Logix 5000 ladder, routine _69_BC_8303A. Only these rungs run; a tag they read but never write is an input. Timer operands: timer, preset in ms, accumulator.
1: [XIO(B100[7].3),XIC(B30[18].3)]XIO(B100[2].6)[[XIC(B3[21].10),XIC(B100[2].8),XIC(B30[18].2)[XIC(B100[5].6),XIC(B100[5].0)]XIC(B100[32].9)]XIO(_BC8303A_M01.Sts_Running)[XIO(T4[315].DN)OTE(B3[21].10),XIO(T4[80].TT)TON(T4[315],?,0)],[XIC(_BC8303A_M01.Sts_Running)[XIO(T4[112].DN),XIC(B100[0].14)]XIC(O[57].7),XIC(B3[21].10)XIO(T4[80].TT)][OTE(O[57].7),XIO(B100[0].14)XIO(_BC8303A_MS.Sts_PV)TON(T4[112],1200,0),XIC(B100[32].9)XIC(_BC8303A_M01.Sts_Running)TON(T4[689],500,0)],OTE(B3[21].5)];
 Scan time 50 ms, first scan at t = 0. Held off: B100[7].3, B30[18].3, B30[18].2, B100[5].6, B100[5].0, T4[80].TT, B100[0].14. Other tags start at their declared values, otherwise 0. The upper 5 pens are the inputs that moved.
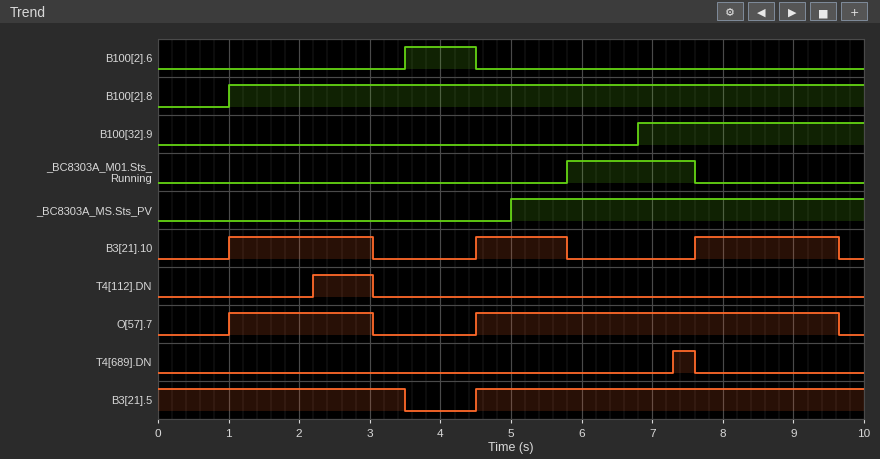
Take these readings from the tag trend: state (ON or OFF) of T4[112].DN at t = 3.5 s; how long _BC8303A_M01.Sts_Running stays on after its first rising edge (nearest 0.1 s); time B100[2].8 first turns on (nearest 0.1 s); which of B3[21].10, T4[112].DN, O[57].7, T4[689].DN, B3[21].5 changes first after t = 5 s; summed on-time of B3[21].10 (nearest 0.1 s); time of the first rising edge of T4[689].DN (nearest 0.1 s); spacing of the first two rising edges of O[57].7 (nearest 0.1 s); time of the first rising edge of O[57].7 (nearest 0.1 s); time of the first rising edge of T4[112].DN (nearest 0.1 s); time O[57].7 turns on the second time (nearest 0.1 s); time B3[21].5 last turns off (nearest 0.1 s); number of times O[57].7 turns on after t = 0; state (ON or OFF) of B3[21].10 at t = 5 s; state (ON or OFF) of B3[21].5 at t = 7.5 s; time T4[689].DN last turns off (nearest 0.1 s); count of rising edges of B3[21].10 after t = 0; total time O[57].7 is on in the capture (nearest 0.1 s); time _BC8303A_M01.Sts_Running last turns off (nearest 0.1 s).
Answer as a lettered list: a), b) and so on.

a) OFF
b) 1.8 s
c) 1.0 s
d) B3[21].10
e) 5.4 s
f) 7.3 s
g) 3.5 s
h) 1.0 s
i) 2.2 s
j) 4.5 s
k) 3.5 s
l) 2
m) ON
n) ON
o) 7.6 s
p) 3
q) 7.2 s
r) 7.6 s
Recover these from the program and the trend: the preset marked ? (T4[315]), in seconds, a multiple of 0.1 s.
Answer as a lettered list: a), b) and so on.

a) 2.0 s
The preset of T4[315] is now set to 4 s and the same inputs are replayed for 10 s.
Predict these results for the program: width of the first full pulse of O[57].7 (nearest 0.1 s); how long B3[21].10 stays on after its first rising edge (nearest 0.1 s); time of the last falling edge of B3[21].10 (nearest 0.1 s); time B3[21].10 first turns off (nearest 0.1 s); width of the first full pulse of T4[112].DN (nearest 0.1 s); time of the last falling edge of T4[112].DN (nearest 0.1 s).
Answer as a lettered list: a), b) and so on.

a) 2.5 s
b) 2.5 s
c) 5.8 s
d) 3.5 s
e) 1.3 s
f) 3.5 s
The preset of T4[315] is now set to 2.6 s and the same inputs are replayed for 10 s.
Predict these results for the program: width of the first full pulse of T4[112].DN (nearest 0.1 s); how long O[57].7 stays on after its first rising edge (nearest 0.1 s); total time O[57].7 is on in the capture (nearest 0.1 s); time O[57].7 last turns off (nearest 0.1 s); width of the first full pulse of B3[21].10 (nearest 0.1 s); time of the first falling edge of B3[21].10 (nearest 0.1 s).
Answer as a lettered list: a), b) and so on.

a) 1.3 s
b) 2.5 s
c) 8.0 s
d) 3.5 s
e) 2.5 s
f) 3.5 s
